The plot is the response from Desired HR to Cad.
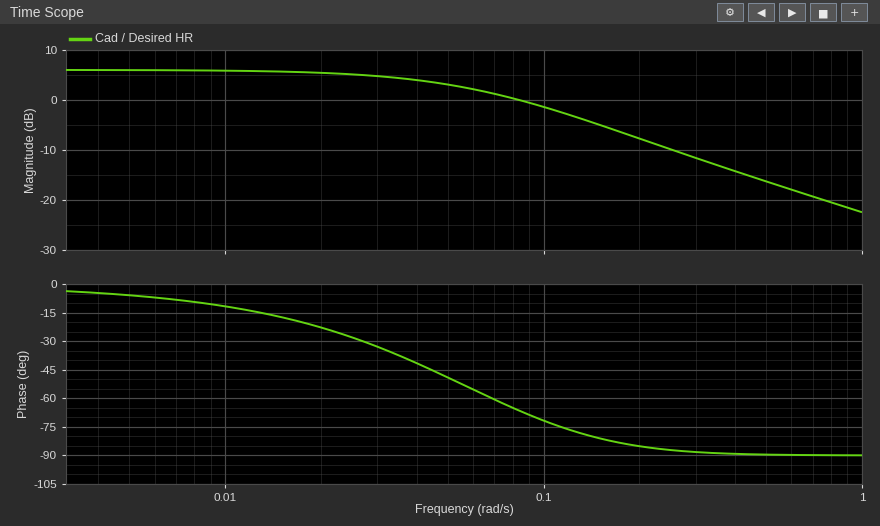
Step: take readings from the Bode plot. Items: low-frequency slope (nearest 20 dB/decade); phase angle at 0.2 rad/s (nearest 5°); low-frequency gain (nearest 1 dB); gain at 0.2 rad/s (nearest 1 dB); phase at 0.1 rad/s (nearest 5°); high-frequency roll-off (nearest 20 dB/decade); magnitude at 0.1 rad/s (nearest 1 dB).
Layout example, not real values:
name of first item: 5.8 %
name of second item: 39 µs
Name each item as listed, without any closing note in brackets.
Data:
low-frequency slope: 0 dB/decade
phase angle at 0.2 rad/s: -85°
low-frequency gain: 6 dB
gain at 0.2 rad/s: -8 dB
phase at 0.1 rad/s: -70°
high-frequency roll-off: -20 dB/decade
magnitude at 0.1 rad/s: -1 dB
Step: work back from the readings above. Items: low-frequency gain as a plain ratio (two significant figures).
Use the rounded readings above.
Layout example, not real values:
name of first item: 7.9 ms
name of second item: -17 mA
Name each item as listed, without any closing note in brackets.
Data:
low-frequency gain as a plain ratio: 2.0
